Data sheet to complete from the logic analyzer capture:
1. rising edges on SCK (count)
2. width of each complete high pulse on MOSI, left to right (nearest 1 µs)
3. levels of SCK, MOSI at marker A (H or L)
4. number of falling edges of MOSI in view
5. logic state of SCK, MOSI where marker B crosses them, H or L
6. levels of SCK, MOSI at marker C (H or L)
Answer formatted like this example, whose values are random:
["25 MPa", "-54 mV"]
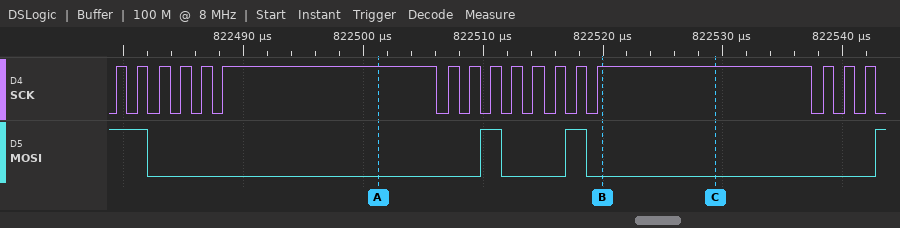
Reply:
["17", "2 µs, 2 µs", "SCK=H, MOSI=L", "3", "SCK=H, MOSI=L", "SCK=H, MOSI=L"]
